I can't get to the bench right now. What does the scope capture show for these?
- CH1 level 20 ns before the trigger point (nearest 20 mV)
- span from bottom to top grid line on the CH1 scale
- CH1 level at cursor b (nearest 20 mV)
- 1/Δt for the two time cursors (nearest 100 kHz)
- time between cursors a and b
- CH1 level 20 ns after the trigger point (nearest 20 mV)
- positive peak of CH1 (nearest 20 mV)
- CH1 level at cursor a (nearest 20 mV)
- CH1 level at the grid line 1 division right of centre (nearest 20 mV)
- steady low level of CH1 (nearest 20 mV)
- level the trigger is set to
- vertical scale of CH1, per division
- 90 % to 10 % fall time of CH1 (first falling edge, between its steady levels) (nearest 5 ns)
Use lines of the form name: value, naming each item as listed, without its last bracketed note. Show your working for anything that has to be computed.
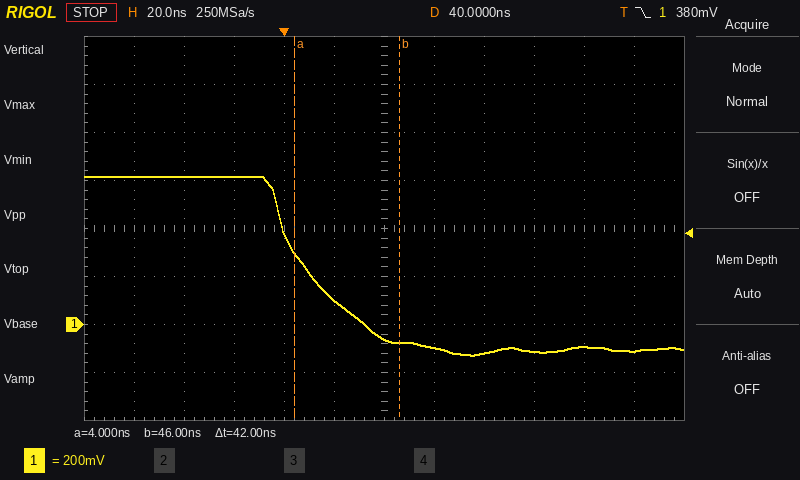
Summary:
CH1 level 20 ns before the trigger point: 620 mV
span from bottom to top grid line on the CH1 scale: 1.6 V
CH1 level at cursor b: -80 mV
1/Δt for the two time cursors: 1 / 42 ns ≈ 23.8 MHz
time between cursors a and b: 42 ns
CH1 level 20 ns after the trigger point: 100 mV
positive peak of CH1: 620 mV
CH1 level at cursor a: 300 mV
CH1 level at the grid line 1 division right of centre: -100 mV
steady low level of CH1: -100 mV
level the trigger is set to: 380 mV
vertical scale of CH1, per division: 200 mV
90 % to 10 % fall time of CH1 (first falling edge, between its steady levels): 40 ns
